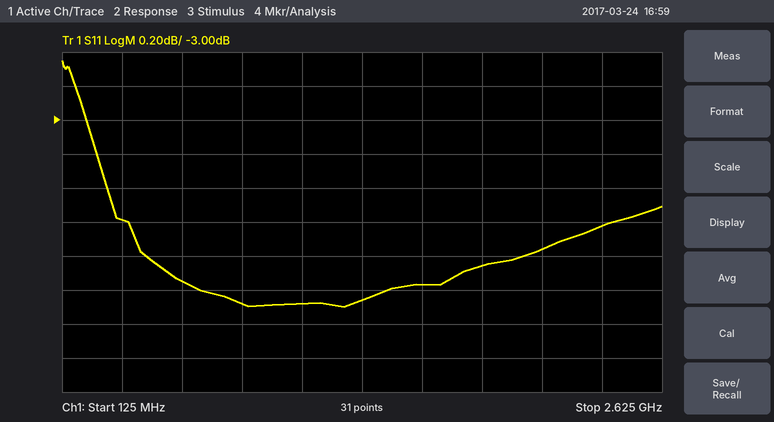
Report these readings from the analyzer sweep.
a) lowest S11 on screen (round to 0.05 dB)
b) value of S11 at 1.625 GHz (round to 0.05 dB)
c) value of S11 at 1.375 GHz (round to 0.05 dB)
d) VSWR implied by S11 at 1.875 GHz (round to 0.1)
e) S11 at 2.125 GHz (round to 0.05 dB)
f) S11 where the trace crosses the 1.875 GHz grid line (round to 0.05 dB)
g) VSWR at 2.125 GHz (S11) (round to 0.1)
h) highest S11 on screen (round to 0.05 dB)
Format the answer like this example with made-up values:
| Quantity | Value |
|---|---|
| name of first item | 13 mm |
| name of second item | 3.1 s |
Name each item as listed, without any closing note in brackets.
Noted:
| Quantity | Value |
|---|---|
| lowest S11 on screen | -4.10 dB |
| value of S11 at 1.625 GHz | -3.95 dB |
| value of S11 at 1.375 GHz | -4.05 dB |
| VSWR implied by S11 at 1.875 GHz | 4.6 |
| S11 at 2.125 GHz | -3.75 dB |
| S11 where the trace crosses the 1.875 GHz grid line | -3.85 dB |
| VSWR at 2.125 GHz (S11) | 4.7 |
| highest S11 on screen | -2.65 dB |
